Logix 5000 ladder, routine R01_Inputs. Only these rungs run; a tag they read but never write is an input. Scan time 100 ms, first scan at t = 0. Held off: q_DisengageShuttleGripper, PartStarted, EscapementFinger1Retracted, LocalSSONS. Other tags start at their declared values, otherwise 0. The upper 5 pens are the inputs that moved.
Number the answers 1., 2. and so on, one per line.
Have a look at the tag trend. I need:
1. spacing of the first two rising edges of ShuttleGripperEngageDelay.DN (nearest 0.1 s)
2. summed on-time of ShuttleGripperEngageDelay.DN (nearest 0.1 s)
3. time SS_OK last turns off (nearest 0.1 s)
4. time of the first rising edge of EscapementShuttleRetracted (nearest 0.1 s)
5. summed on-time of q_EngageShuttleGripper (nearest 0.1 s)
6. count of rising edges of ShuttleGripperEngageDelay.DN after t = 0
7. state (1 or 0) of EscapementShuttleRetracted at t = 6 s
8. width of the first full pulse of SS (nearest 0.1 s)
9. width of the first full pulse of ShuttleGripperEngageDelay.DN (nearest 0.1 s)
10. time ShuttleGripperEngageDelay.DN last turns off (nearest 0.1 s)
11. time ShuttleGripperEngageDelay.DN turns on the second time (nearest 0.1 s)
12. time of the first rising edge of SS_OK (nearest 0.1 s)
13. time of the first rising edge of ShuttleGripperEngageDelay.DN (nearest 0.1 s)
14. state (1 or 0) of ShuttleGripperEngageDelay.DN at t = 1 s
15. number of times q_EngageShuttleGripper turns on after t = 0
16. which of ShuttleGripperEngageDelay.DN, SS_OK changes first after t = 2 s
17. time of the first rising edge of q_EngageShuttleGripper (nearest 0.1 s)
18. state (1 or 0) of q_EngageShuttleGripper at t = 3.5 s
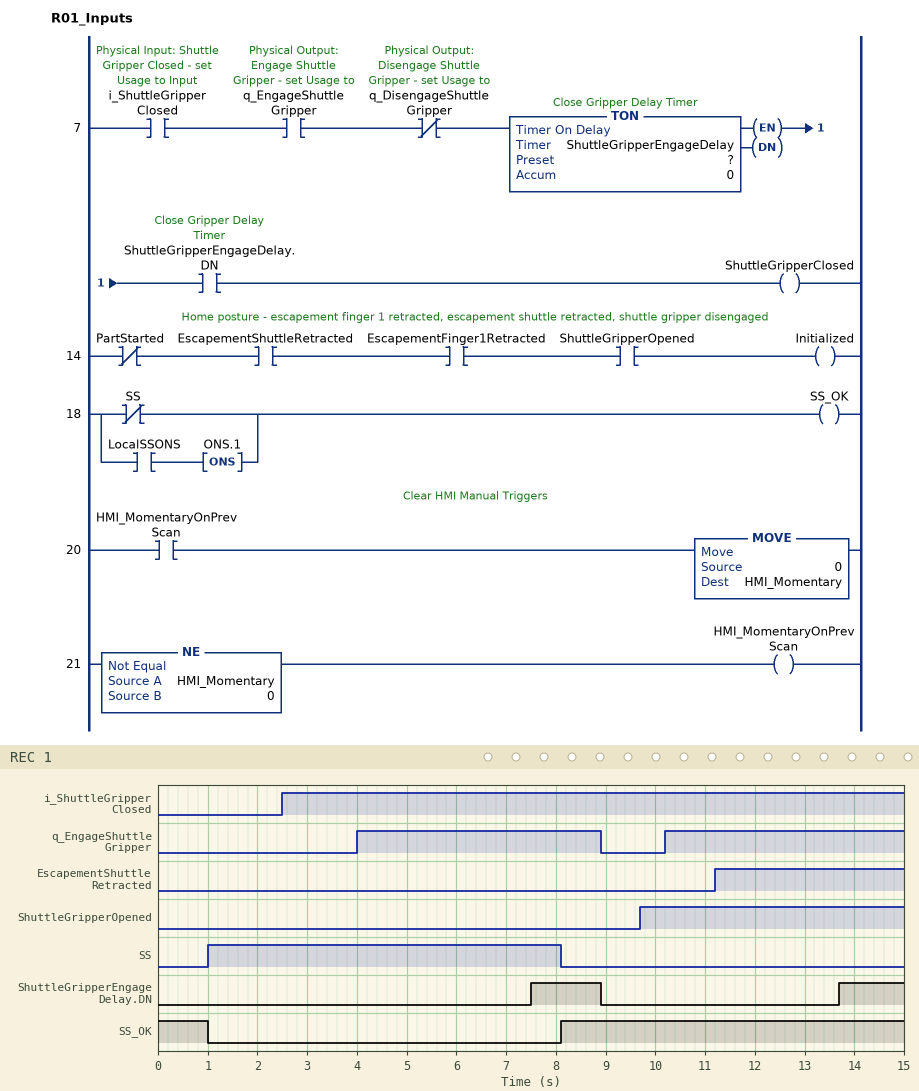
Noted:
1. 6.2 s
2. 2.7 s
3. 1.0 s
4. 11.2 s
5. 9.7 s
6. 2
7. 0
8. 7.1 s
9. 1.4 s
10. 8.9 s
11. 13.7 s
12. 8.1 s
13. 7.5 s
14. 0
15. 2
16. ShuttleGripperEngageDelay.DN
17. 4.0 s
18. 0
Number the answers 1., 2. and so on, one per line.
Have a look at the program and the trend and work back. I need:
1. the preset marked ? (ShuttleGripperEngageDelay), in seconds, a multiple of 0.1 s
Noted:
1. 3.5 s
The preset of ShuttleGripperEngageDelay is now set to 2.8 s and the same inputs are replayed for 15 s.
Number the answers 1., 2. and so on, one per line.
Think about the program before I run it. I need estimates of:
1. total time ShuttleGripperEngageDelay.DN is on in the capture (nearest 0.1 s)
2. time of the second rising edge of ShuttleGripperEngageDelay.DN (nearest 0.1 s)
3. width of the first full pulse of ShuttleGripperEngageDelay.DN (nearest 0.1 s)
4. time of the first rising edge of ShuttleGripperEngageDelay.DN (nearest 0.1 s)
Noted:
1. 4.1 s
2. 13.0 s
3. 2.1 s
4. 6.8 s
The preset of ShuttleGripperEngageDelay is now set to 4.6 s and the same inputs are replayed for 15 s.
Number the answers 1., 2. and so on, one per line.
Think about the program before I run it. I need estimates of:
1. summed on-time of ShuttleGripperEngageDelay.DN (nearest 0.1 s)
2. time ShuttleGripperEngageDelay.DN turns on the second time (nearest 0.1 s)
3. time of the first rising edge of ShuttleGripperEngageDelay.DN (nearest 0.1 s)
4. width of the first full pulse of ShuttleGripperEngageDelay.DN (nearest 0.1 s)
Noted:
1. 0.5 s
2. 14.8 s
3. 8.6 s
4. 0.3 s
